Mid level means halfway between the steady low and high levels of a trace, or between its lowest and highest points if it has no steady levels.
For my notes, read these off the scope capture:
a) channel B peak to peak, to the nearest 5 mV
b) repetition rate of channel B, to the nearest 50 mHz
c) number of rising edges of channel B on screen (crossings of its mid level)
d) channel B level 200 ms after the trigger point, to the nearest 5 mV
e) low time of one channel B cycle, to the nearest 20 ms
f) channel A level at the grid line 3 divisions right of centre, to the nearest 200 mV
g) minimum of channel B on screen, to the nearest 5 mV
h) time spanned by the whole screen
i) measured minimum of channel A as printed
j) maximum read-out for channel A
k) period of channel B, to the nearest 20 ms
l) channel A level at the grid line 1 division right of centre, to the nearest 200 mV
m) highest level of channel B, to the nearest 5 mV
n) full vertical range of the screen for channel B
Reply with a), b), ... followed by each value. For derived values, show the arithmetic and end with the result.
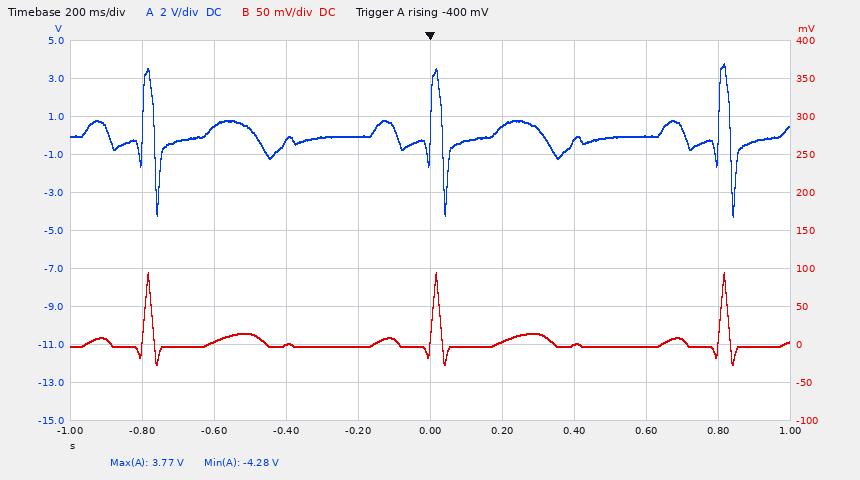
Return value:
a) 95 mV − (-25 mV) = 120 mV
b) 1 / 800 ms ≈ 1.25 Hz
c) 3
d) 5 mV
e) 780 ms
f) 0.0 V
g) -25 mV
h) 2 s
i) -4.28 V
j) 3.77 V
k) 800 ms
l) 400 mV
m) 95 mV
n) 500 mV
